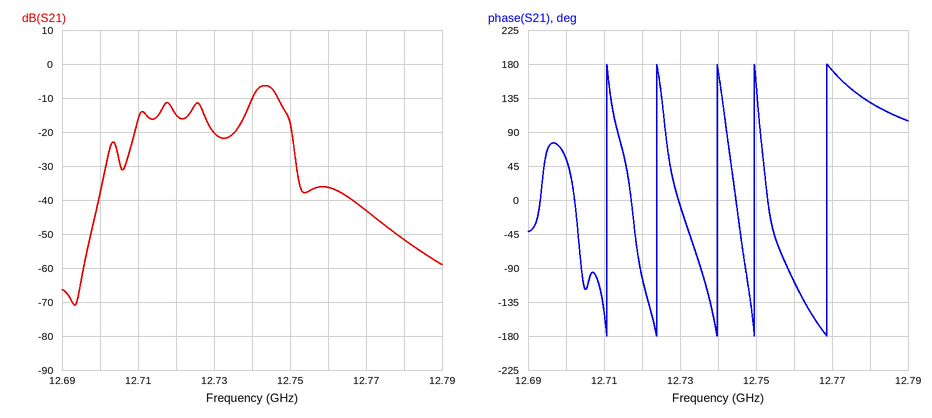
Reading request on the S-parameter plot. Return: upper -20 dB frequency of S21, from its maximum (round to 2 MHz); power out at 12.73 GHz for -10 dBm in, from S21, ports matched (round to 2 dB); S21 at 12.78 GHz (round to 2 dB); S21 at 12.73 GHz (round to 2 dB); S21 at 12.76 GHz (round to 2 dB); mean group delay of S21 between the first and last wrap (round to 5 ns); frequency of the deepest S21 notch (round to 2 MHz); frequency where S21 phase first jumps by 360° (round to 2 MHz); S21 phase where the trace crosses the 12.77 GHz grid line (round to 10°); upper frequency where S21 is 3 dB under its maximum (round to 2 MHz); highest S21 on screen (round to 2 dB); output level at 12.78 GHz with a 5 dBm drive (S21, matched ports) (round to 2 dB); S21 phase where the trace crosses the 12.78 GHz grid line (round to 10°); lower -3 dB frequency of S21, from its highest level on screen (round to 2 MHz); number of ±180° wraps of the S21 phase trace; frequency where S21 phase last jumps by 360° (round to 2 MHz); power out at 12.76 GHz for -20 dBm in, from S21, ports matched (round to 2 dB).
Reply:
12.752 GHz
-30 dBm
-52 dB
-20 dB
-36 dB
70 ns
12.694 GHz
12.710 GHz
170°
12.746 GHz
-6 dB
-46 dBm
130°
12.740 GHz
5
12.768 GHz
-56 dBm
